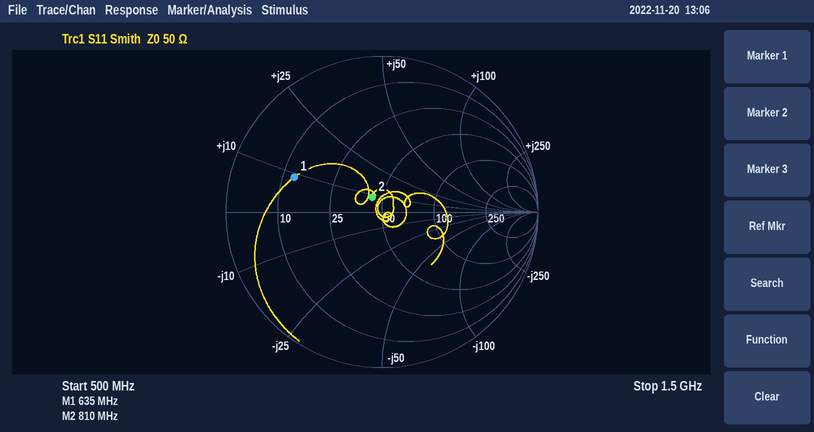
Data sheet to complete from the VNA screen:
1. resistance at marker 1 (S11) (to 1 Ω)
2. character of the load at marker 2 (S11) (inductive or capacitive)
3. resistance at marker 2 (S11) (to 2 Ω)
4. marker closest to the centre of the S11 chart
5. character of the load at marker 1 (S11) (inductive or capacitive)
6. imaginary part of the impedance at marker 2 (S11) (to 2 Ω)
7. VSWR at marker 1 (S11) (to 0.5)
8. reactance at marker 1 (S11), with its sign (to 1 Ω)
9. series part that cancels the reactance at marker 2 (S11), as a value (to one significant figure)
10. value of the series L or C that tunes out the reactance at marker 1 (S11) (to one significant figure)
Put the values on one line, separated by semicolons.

13 Ω; inductive; 44 Ω; marker 2; inductive; +8 Ω; 4.0; +9 Ω; 20 pF; 30 pF
